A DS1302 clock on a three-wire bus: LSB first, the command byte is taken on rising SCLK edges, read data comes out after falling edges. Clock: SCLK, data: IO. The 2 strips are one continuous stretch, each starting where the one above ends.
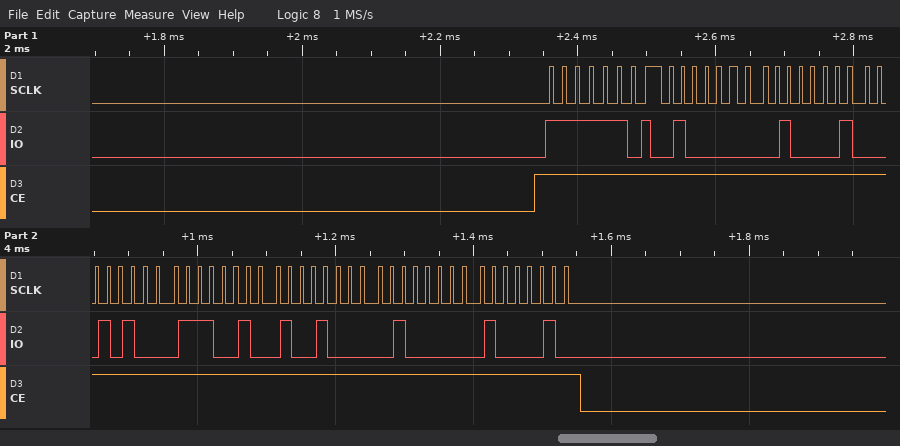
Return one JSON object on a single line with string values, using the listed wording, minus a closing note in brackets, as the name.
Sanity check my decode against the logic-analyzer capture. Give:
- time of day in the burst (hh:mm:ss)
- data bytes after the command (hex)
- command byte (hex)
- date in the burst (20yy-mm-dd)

{"time of day in the burst": "14:42:02", "data bytes after the command": "02 42 14 27 09 02 21", "command byte": "0xBF", "date in the burst": "2021-09-27"}
